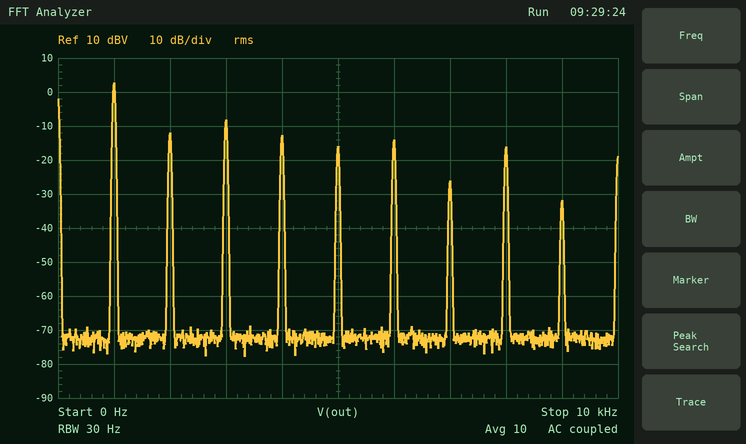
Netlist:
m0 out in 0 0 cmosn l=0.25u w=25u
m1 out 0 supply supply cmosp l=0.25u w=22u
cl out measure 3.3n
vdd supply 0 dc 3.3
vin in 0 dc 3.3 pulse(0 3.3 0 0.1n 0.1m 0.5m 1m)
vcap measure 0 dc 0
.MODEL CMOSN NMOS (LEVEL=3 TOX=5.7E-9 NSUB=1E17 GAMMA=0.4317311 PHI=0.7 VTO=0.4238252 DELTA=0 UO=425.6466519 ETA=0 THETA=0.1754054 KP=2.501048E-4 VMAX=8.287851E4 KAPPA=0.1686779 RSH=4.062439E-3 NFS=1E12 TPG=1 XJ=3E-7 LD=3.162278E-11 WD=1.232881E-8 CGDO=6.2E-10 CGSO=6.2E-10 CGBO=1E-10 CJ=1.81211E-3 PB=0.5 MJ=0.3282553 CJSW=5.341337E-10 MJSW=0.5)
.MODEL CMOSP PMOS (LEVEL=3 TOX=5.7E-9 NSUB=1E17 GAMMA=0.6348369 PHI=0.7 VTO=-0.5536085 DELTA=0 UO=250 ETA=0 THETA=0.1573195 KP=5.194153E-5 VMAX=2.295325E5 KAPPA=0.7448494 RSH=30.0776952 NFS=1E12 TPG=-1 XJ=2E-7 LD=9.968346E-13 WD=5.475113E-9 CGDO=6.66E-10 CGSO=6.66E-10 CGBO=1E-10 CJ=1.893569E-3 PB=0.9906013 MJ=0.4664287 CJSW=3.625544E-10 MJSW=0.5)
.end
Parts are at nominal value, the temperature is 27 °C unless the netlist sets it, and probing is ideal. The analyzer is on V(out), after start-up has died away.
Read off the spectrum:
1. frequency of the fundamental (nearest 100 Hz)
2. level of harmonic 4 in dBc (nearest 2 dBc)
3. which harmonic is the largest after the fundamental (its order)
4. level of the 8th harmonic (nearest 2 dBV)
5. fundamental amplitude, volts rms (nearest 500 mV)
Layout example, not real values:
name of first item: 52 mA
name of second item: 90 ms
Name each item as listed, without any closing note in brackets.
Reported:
frequency of the fundamental: 1.0 kHz
level of harmonic 4 in dBc: -16 dBc
which harmonic is the largest after the fundamental: 3
level of the 8th harmonic: -16 dBV
fundamental amplitude, volts rms: 1.5 V
